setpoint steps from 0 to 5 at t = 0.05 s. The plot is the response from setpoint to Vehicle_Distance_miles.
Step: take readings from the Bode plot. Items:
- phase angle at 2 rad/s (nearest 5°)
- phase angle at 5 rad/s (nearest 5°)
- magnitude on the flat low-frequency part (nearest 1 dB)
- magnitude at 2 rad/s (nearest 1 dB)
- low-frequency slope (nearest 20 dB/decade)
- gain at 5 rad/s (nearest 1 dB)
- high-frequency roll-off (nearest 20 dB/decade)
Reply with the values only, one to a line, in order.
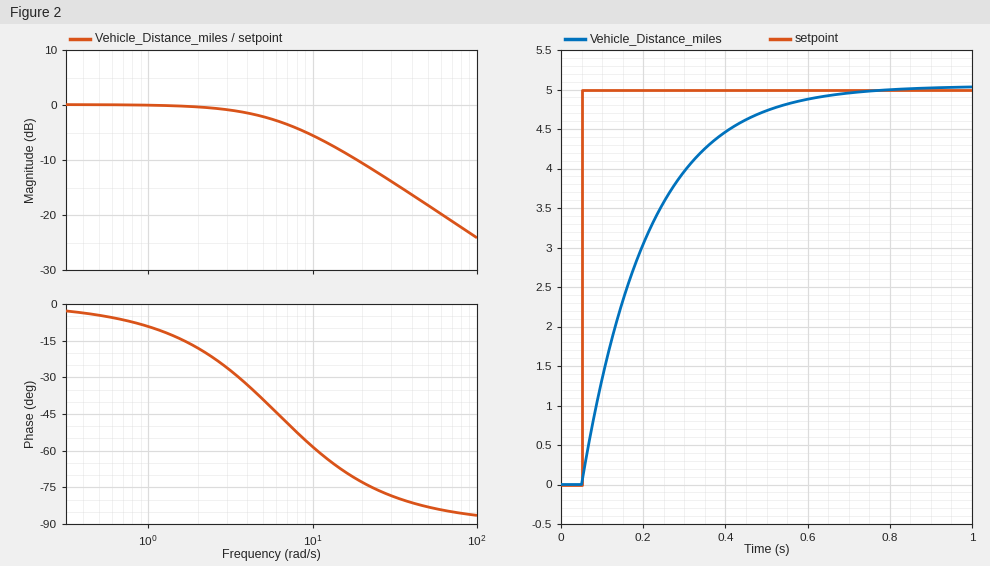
-20°
-40°
0 dB
0 dB
0 dB/decade
-2 dB
-20 dB/decade
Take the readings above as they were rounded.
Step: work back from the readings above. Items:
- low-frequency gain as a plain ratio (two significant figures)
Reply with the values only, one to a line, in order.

1.0
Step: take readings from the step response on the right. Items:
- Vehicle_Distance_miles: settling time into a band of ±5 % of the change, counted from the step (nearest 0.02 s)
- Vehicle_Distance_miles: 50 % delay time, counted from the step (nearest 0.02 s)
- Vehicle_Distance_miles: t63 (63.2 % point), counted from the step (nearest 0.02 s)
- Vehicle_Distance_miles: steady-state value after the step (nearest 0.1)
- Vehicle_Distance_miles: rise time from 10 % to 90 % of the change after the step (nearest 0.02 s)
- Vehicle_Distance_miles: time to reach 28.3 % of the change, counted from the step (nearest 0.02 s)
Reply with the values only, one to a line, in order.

0.48 s
0.12 s
0.16 s
5.0
0.36 s
0.06 s
